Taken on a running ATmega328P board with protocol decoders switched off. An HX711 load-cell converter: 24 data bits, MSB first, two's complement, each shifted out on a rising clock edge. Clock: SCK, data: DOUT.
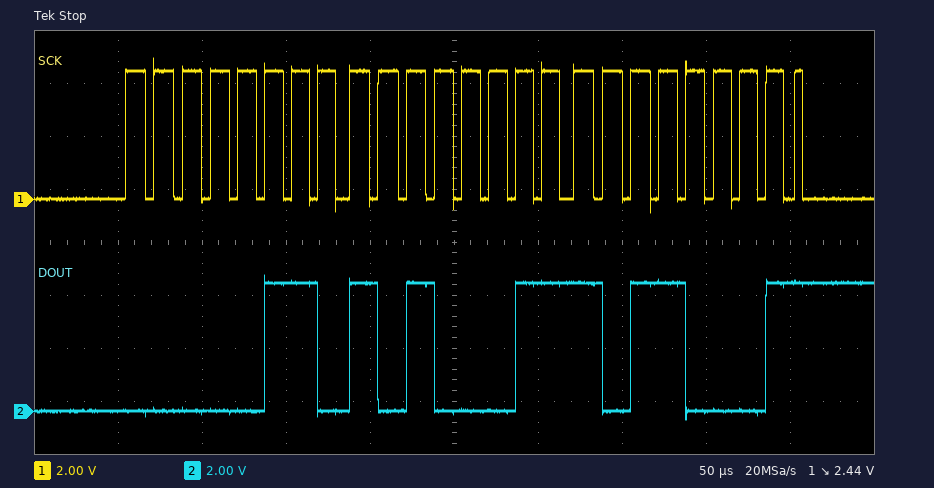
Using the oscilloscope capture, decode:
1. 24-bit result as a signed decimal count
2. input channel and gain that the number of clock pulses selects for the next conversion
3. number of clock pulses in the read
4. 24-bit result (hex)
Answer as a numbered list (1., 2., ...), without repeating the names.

1. 435121
2. channel A, gain 128
3. 25
4. 0x06A3B1
